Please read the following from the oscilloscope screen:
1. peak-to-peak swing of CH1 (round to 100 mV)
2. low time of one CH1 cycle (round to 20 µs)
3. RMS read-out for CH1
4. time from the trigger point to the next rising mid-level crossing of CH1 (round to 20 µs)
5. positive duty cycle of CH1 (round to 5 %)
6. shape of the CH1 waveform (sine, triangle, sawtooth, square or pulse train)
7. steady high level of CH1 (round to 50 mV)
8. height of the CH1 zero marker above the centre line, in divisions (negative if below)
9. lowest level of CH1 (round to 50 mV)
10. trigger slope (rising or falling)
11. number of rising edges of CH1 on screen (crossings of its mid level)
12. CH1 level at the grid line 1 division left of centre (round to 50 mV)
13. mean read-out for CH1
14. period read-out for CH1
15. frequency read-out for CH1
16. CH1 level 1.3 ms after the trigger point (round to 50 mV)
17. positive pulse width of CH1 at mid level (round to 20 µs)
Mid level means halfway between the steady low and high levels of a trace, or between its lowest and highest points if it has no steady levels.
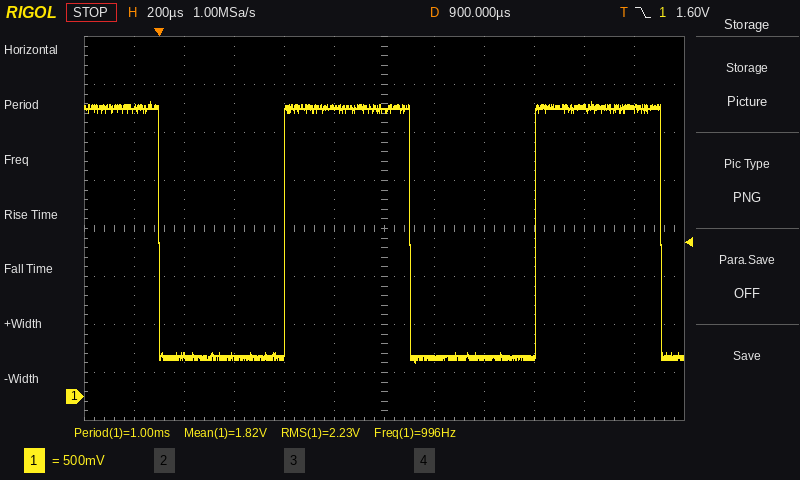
2.70 V
500 µs
2.23 V
500 µs
50 %
square
3.00 V
-3.5 div
350 mV
falling
2
3.00 V
1.82 V
1.00 ms
996 Hz
400 mV
500 µs
